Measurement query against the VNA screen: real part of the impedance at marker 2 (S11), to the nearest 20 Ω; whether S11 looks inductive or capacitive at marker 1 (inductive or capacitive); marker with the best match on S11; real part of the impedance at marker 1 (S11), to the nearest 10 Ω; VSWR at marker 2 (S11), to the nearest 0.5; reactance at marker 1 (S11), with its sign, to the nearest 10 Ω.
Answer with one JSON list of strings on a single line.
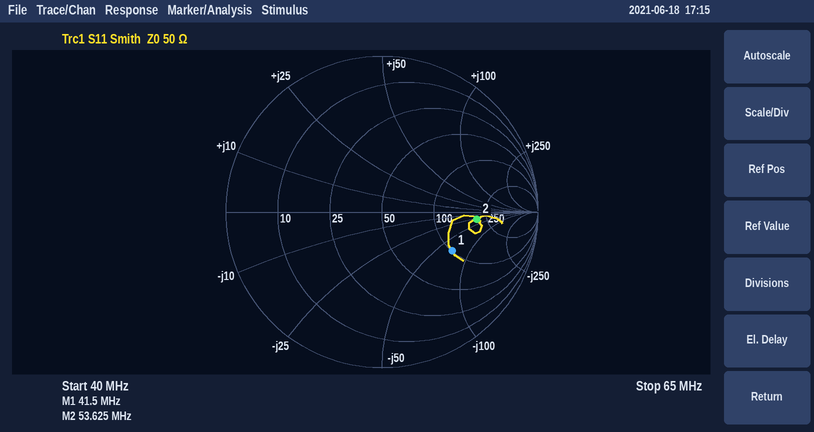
["200 Ω", "capacitive", "marker 1", "100 Ω", "4.0", "-70 Ω"]
